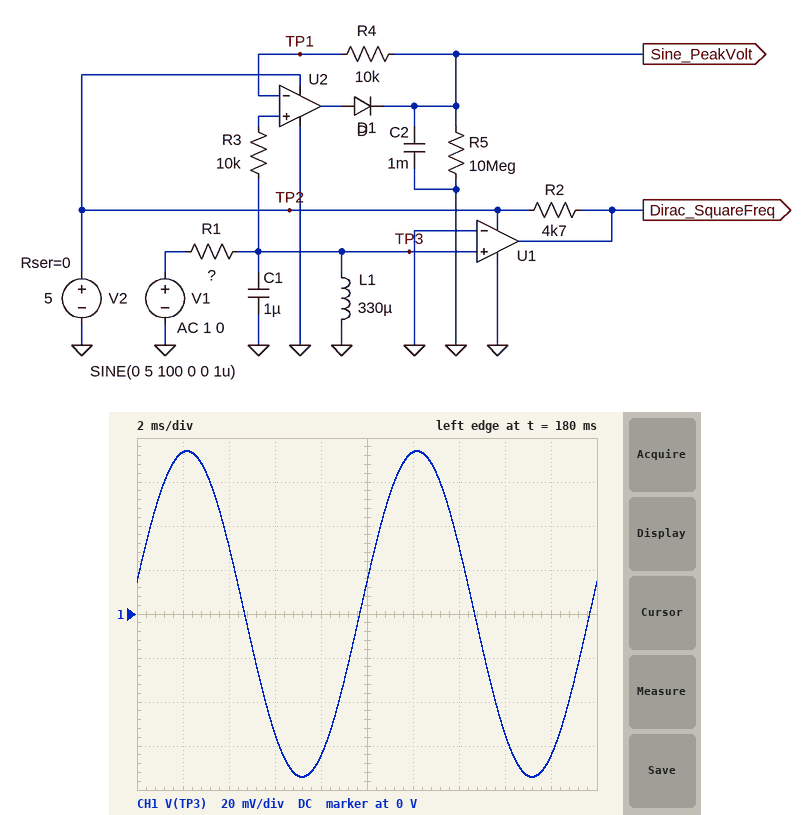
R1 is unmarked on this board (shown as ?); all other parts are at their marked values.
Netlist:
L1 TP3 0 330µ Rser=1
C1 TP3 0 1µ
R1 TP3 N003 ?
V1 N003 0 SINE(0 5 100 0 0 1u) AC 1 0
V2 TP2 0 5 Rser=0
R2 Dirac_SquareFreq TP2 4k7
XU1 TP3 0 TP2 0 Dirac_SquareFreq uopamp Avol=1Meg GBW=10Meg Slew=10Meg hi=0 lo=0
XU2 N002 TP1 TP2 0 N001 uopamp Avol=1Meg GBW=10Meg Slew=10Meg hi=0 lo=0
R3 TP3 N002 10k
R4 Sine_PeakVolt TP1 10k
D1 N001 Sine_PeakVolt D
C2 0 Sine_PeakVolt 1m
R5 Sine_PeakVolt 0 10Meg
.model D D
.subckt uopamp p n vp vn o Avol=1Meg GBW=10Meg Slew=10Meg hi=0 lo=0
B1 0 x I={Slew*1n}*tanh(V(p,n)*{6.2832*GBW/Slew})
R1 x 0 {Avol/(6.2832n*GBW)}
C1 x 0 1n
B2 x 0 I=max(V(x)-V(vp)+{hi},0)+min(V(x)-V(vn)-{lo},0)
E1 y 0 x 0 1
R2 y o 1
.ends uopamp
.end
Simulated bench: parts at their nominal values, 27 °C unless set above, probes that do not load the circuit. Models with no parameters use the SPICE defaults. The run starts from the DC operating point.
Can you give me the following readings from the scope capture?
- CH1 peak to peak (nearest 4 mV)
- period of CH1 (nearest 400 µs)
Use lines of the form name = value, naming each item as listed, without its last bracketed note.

CH1 peak to peak = 148 mV
period of CH1 = 10.0 ms
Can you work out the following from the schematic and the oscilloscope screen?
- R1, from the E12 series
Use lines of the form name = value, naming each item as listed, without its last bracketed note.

R1, from the E12 series = 68 Ω
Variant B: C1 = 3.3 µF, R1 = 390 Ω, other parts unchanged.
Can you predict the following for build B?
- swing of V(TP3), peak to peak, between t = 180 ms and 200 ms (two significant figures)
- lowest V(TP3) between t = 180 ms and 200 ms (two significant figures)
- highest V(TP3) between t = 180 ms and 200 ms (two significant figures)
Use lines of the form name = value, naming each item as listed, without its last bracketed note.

swing of V(TP3), peak to peak, between t = 180 ms and 200 ms = 26 mV
lowest V(TP3) between t = 180 ms and 200 ms = -13 mV
highest V(TP3) between t = 180 ms and 200 ms = 13 mV
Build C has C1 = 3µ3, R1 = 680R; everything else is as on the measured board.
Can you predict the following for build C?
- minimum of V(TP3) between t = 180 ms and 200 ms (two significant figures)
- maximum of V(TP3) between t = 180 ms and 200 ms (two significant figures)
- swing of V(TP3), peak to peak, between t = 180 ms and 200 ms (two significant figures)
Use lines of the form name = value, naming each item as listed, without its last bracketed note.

minimum of V(TP3) between t = 180 ms and 200 ms = -7.5 mV
maximum of V(TP3) between t = 180 ms and 200 ms = 7.5 mV
swing of V(TP3), peak to peak, between t = 180 ms and 200 ms = 15 mV
